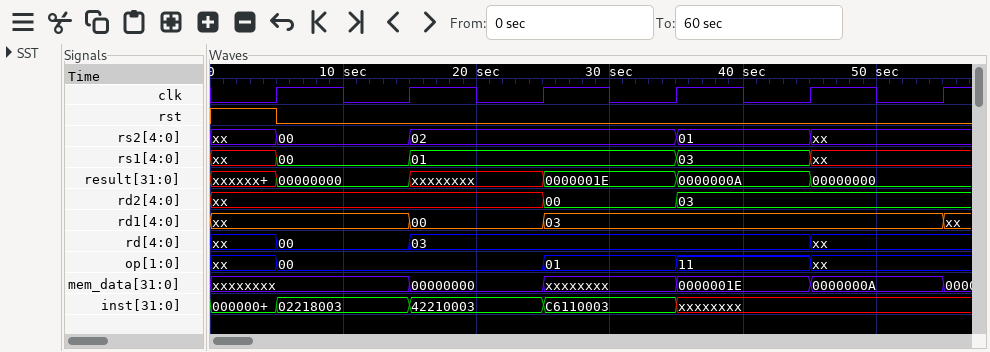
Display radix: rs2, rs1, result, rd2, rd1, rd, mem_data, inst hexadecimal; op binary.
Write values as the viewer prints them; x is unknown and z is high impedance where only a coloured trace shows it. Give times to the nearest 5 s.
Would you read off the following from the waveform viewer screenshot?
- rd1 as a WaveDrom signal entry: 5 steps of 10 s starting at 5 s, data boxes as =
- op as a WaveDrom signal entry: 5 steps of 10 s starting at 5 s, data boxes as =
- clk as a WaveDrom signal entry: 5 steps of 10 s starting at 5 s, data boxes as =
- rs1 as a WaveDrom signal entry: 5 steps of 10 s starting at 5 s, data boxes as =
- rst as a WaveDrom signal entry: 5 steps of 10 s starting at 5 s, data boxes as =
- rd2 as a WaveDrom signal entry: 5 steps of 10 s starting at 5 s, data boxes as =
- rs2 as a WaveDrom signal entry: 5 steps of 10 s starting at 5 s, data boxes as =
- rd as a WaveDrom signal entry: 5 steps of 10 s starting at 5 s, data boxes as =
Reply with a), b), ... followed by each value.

a) {name: 'rd1', wave: 'x==..', data: '00 03'}
b) {name: 'op', wave: '=.==x', data: '00 01 11'}
c) {name: 'clk', wave: 'p....'}
d) {name: 'rs1', wave: '==.=x', data: '00 01 03'}
e) {name: 'rst', wave: '0....'}
f) {name: 'rd2', wave: 'x.==.', data: '00 03'}
g) {name: 'rs2', wave: '==.=x', data: '00 02 01'}
h) {name: 'rd', wave: '==..x', data: '00 03'}
